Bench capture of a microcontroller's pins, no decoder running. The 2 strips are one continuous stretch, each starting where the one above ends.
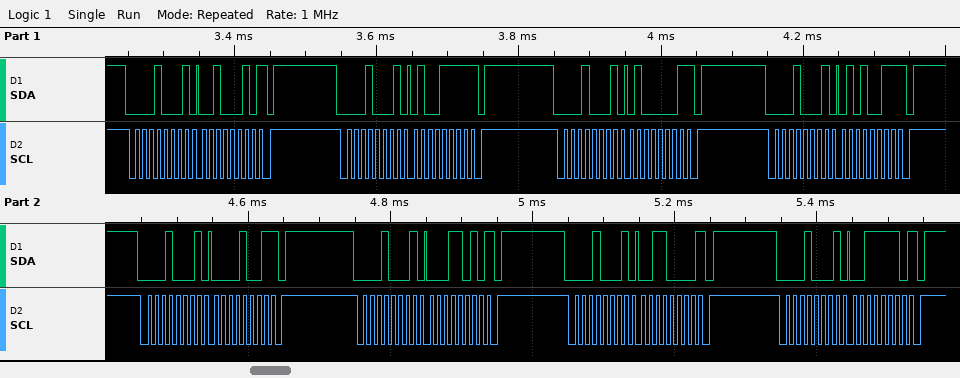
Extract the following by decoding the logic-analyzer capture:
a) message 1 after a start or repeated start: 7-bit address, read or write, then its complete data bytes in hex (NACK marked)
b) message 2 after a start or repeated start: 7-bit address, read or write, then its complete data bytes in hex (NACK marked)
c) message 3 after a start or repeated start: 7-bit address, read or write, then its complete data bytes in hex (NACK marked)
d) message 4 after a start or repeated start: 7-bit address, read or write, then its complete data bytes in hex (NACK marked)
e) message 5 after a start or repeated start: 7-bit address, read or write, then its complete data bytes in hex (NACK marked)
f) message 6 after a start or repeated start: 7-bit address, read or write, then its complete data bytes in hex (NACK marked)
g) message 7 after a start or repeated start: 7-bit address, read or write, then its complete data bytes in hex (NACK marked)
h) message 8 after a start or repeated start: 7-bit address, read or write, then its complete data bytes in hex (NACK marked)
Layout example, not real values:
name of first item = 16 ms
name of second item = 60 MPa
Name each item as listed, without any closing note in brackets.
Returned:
message 1 after a start or repeated start: 7-bit address, read or write, then its complete data bytes in hex = 0x08 read: 22 NACK
message 2 after a start or repeated start: 7-bit address, read or write, then its complete data bytes in hex = 0x08 read: 4F NACK
message 3 after a start or repeated start: 7-bit address, read or write, then its complete data bytes in hex = 0x08 read: 41 NACK
message 4 after a start or repeated start: 7-bit address, read or write, then its complete data bytes in hex = 0x08 read: 53 NACK
message 5 after a start or repeated start: 7-bit address, read or write, then its complete data bytes in hex = 0x08 read: 09 NACK
message 6 after a start or repeated start: 7-bit address, read or write, then its complete data bytes in hex = 0x08 read: 1A NACK
message 7 after a start or repeated start: 7-bit address, read or write, then its complete data bytes in hex = 0x08 read: 30 NACK
message 8 after a start or repeated start: 7-bit address, read or write, then its complete data bytes in hex = 0x08 read: 3E NACK
